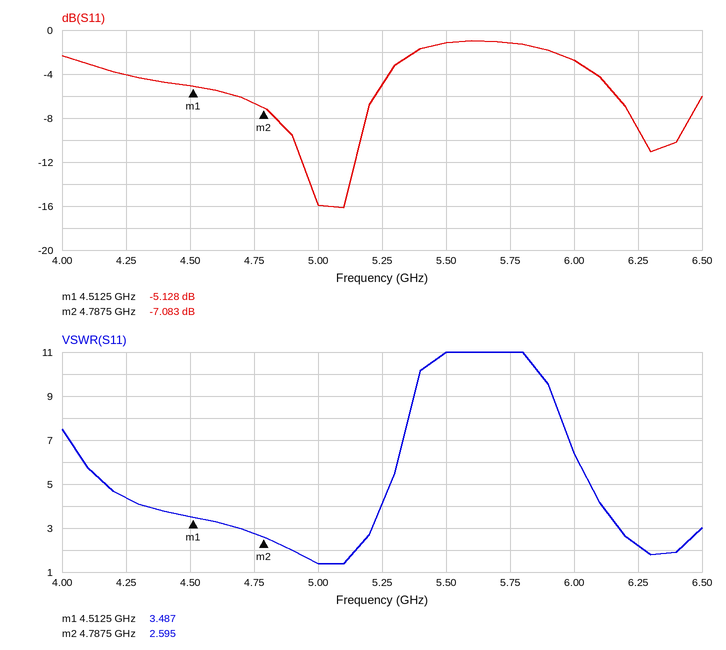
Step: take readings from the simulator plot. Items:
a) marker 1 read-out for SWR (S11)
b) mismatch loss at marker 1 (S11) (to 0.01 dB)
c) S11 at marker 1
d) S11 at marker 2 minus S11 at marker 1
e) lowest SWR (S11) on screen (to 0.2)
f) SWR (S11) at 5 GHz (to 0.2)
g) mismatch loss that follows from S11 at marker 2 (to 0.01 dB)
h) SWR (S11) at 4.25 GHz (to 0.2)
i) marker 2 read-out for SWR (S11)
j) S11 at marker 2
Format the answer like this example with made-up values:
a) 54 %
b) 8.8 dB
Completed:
a) 3.487
b) 1.59 dB
c) -5.128 dB
d) -1.955 dB
e) 1.4
f) 1.4
g) 0.95 dB
h) 4.4
i) 2.595
j) -7.083 dB
